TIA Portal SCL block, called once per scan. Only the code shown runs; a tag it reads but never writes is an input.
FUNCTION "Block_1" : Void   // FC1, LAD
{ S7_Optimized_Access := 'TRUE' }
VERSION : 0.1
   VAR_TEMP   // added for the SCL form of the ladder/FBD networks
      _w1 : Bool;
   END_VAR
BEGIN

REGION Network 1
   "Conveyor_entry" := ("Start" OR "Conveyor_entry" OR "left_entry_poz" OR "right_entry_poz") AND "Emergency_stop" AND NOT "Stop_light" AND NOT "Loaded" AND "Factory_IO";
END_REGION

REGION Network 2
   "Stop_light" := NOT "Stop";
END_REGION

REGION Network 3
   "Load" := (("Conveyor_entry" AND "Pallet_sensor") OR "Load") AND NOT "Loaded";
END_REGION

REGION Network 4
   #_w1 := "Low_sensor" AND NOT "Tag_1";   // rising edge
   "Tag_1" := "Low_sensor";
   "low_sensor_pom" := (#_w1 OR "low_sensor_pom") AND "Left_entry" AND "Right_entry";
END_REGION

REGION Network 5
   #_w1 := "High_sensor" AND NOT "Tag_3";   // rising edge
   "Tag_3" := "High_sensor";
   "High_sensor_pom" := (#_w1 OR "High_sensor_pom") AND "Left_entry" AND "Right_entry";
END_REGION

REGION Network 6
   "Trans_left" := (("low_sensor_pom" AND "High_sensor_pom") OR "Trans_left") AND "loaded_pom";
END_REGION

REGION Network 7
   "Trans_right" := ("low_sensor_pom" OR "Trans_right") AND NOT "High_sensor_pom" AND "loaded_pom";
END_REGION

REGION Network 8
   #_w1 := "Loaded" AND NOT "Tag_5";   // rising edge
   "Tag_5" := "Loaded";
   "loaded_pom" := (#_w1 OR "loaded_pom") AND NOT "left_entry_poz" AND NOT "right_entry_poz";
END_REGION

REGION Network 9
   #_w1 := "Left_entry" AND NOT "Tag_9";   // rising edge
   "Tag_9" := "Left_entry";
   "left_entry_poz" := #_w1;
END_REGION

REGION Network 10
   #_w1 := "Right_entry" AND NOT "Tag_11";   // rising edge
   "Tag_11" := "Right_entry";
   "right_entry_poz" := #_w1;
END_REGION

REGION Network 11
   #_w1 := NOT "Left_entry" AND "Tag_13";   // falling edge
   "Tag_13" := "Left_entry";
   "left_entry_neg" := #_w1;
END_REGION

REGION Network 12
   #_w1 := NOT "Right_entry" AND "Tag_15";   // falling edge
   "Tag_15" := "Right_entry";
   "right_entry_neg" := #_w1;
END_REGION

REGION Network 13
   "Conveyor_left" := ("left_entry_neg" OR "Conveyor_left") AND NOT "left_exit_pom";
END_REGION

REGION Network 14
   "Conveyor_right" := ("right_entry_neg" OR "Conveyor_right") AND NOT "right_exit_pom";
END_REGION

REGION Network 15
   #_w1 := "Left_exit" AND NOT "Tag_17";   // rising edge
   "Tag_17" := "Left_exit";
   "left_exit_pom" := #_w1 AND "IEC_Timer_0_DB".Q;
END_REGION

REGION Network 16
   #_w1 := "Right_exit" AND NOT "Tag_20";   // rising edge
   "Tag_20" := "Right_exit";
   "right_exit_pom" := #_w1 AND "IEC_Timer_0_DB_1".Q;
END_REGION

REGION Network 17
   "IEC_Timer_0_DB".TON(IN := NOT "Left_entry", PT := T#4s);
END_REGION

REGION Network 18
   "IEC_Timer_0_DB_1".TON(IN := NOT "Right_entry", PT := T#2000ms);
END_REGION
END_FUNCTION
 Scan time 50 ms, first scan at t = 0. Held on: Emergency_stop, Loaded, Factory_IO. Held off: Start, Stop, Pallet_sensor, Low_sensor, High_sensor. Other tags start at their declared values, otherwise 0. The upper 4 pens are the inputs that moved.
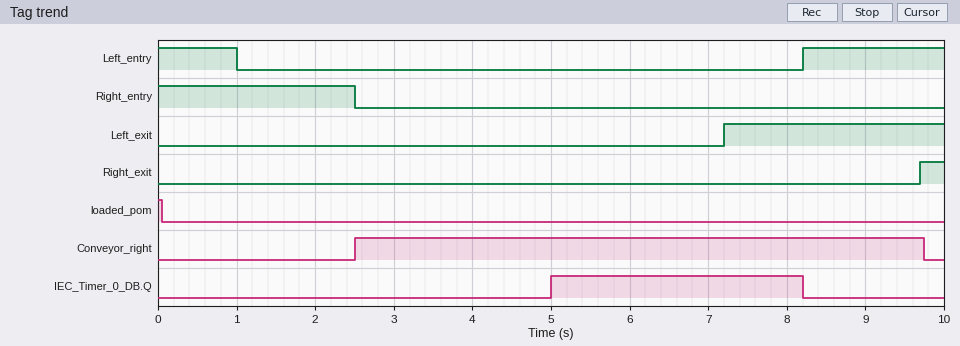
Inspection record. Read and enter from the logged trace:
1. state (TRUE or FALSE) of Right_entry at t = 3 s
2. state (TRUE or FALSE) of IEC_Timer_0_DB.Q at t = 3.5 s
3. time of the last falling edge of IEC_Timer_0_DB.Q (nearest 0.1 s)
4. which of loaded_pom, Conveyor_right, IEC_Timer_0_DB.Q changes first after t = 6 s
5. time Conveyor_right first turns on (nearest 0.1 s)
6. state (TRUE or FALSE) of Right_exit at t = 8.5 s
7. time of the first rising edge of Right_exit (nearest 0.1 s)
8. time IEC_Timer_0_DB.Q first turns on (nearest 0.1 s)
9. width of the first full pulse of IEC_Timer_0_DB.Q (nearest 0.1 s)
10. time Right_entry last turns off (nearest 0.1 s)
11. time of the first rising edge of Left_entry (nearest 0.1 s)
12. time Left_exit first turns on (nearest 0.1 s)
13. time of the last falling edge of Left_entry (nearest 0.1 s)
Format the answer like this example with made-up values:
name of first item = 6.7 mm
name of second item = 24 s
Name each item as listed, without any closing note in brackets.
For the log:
state (TRUE or FALSE) of Right_entry at t = 3 s = FALSE
state (TRUE or FALSE) of IEC_Timer_0_DB.Q at t = 3.5 s = FALSE
time of the last falling edge of IEC_Timer_0_DB.Q = 8.2 s
which of loaded_pom, Conveyor_right, IEC_Timer_0_DB.Q changes first after t = 6 s = IEC_Timer_0_DB.Q
time Conveyor_right first turns on = 2.5 s
state (TRUE or FALSE) of Right_exit at t = 8.5 s = FALSE
time of the first rising edge of Right_exit = 9.7 s
time IEC_Timer_0_DB.Q first turns on = 5.0 s
width of the first full pulse of IEC_Timer_0_DB.Q = 3.2 s
time Right_entry last turns off = 2.5 s
time of the first rising edge of Left_entry = 8.2 s
time Left_exit first turns on = 7.2 s
time of the last falling edge of Left_entry = 1.0 s
